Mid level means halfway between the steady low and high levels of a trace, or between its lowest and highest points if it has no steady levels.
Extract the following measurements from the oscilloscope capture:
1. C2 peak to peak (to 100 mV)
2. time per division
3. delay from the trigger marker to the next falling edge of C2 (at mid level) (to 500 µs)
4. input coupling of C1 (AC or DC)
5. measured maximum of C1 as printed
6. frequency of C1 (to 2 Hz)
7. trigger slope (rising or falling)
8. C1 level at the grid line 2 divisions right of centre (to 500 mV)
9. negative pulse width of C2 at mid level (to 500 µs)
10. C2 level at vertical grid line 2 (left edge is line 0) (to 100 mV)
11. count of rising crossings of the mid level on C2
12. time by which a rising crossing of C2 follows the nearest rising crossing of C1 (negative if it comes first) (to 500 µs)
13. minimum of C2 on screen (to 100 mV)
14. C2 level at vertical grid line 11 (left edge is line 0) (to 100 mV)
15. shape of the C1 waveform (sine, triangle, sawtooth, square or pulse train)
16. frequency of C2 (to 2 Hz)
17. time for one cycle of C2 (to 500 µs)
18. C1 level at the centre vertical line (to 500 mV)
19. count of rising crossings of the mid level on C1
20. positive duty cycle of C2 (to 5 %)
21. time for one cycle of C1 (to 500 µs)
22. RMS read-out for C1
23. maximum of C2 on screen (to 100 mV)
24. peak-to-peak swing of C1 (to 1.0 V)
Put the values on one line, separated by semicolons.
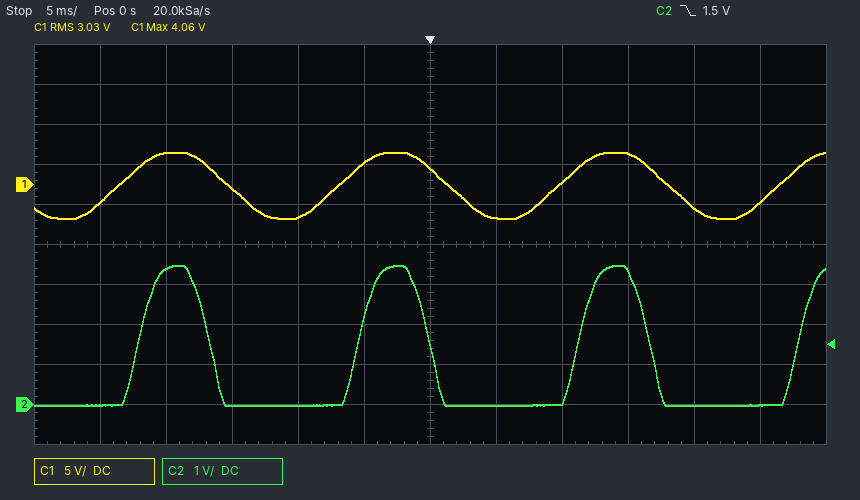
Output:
3.5 V; 5 ms; 16.5 ms; DC; 4.06 V; 60 Hz; falling; 500 mV; 11.5 ms; 3.4 V; 4; +1.5 ms; 0.0 V; 0.0 V; sine; 60 Hz; 16.5 ms; 2.0 V; 4; 30 %; 16.5 ms; 3.03 V; 3.5 V; 8.0 V
